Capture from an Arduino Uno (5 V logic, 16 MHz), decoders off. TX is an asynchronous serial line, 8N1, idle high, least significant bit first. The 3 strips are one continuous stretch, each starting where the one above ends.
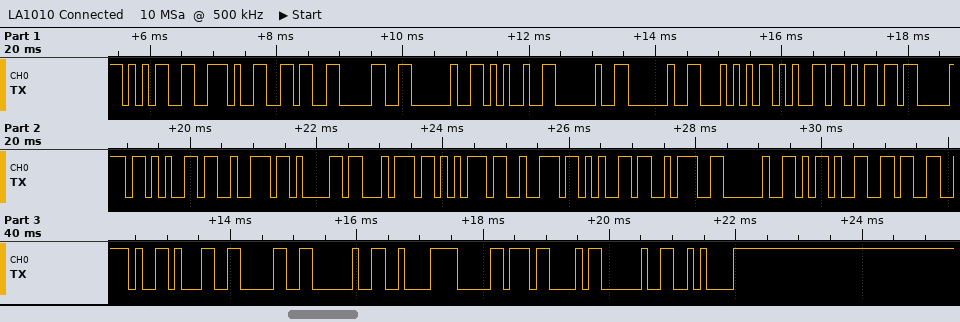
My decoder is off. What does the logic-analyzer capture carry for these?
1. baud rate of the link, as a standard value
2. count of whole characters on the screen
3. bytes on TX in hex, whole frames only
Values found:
9600 baud
32
35 2E 36 30 20 25 20 20 54 65 6D 70 65 72 61 74 75 72 65 3A 20 2D 36 2E 31 30 20 C2 B0 43 20 0A
